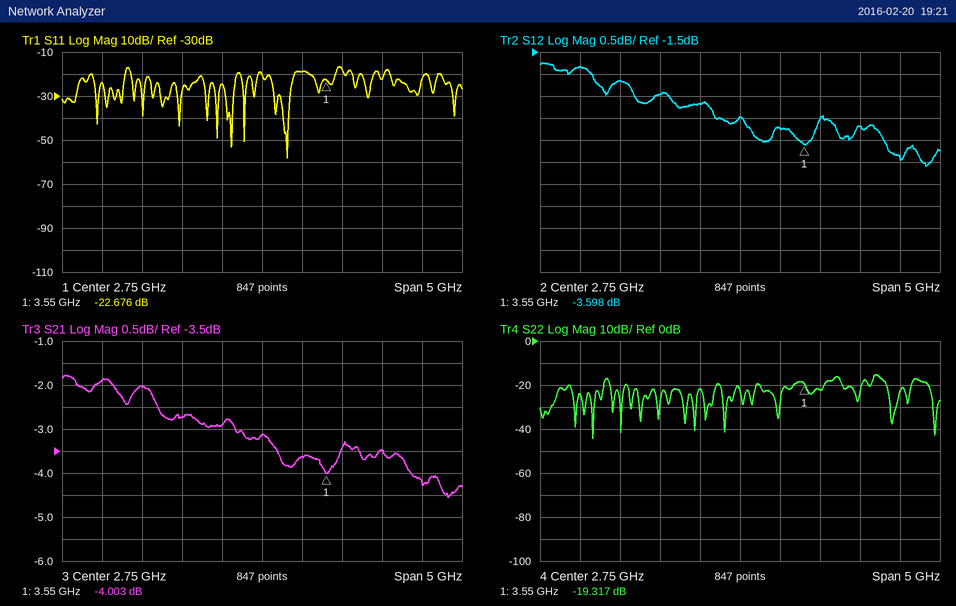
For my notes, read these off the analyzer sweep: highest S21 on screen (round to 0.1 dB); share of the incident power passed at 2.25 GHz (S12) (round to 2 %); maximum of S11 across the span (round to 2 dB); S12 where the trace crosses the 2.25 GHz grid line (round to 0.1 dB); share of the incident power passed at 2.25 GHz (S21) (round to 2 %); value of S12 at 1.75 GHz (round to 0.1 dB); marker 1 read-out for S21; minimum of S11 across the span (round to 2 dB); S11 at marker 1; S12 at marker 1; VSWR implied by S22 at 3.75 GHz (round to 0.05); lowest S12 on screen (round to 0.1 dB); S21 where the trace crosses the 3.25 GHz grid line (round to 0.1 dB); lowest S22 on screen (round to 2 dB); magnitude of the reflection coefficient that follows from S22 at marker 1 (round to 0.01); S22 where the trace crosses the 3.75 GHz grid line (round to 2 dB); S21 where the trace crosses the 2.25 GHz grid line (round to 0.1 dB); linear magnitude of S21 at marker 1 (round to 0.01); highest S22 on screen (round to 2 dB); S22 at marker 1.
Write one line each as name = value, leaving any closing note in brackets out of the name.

highest S21 on screen = -1.8 dB
share of the incident power passed at 2.25 GHz (S12) = 54 %
maximum of S11 across the span = -16 dB
S12 where the trace crosses the 2.25 GHz grid line = -2.7 dB
share of the incident power passed at 2.25 GHz (S21) = 52 %
value of S12 at 1.75 GHz = -2.5 dB
marker 1 read-out for S21 = -4.003 dB
minimum of S11 across the span = -58 dB
S11 at marker 1 = -22.676 dB
S12 at marker 1 = -3.598 dB
VSWR implied by S22 at 3.75 GHz = 1.15
lowest S12 on screen = -4.1 dB
S21 where the trace crosses the 3.25 GHz grid line = -3.6 dB
lowest S22 on screen = -44 dB
magnitude of the reflection coefficient that follows from S22 at marker 1 = 0.11
S22 where the trace crosses the 3.75 GHz grid line = -22 dB
S21 where the trace crosses the 2.25 GHz grid line = -2.9 dB
linear magnitude of S21 at marker 1 = 0.63
highest S22 on screen = -16 dB
S22 at marker 1 = -19.317 dB
